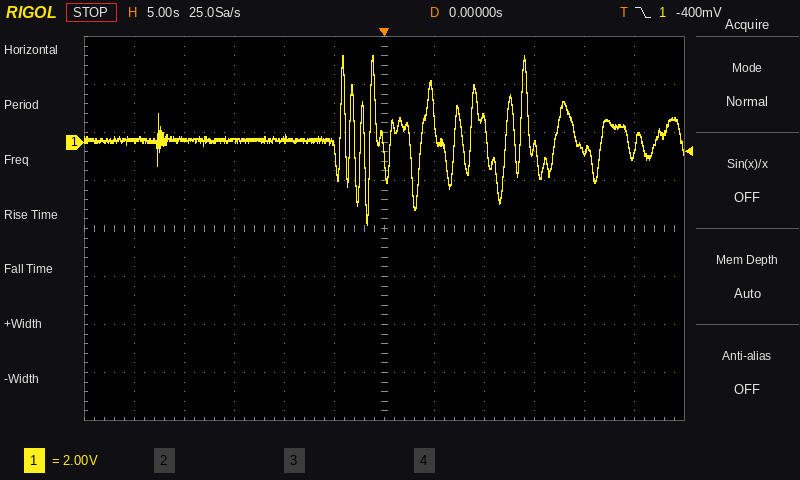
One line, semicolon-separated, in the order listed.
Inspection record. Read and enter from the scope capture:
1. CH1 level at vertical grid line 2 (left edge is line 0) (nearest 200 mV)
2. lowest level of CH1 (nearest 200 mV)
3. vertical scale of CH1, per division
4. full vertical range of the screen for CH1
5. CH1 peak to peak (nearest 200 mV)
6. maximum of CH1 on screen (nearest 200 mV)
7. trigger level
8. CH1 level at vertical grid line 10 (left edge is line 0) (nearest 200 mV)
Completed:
200 mV; -3.4 V; 2 V; 16 V; 7.0 V; 3.6 V; -400 mV; -400 mV
